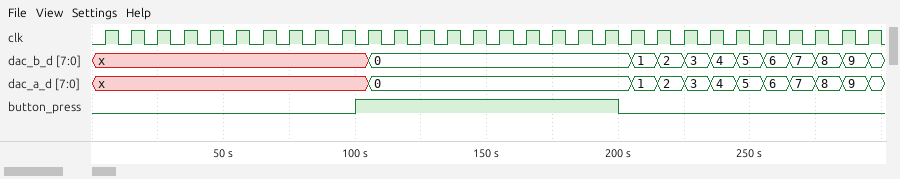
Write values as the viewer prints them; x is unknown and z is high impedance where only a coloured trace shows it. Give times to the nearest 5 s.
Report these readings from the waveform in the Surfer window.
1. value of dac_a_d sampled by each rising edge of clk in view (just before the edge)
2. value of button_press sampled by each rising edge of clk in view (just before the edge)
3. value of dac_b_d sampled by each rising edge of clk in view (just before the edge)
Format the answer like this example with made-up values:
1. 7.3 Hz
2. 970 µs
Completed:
1. x, x, x, x, x, x, x, x, x, x, x, 0, 0, 0, 0, 0, 0, 0, 0, 0, 0, 1, 2, 3, 4, 5, 6, 7, 8, 9
2. 0 0 0 0 0 0 0 0 0 0 1 1 1 1 1 1 1 1 1 1 0 0 0 0 0 0 0 0 0 0
3. x, x, x, x, x, x, x, x, x, x, x, 0, 0, 0, 0, 0, 0, 0, 0, 0, 0, 1, 2, 3, 4, 5, 6, 7, 8, 9
